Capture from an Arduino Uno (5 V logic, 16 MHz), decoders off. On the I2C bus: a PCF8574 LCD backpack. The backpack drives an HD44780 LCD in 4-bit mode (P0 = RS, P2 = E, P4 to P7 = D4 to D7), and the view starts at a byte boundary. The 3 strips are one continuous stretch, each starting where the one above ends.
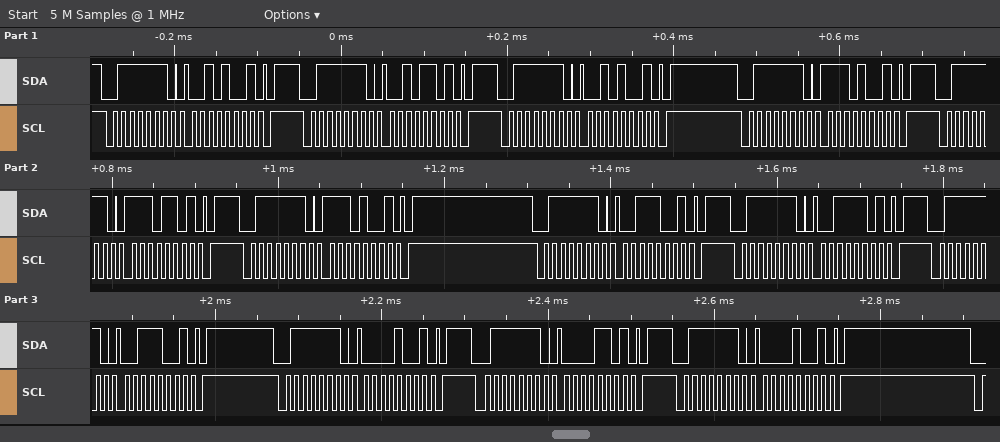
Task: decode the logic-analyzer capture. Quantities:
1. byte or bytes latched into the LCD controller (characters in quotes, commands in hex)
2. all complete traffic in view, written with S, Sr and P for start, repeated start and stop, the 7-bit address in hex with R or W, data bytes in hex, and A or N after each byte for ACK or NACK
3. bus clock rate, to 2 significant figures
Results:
'.' '0'
S 3FW A 29 A P S 3FW A 2D A P S 3FW A 29 A P S 3FW A E9 A P S 3FW A ED A P S 3FW A E9 A P S 3FW A 39 A P S 3FW A 3D A P S 3FW A 39 A P S 3FW A 09 A P S 3FW A 0D A P S 3FW A 09 A P
100 kHz
